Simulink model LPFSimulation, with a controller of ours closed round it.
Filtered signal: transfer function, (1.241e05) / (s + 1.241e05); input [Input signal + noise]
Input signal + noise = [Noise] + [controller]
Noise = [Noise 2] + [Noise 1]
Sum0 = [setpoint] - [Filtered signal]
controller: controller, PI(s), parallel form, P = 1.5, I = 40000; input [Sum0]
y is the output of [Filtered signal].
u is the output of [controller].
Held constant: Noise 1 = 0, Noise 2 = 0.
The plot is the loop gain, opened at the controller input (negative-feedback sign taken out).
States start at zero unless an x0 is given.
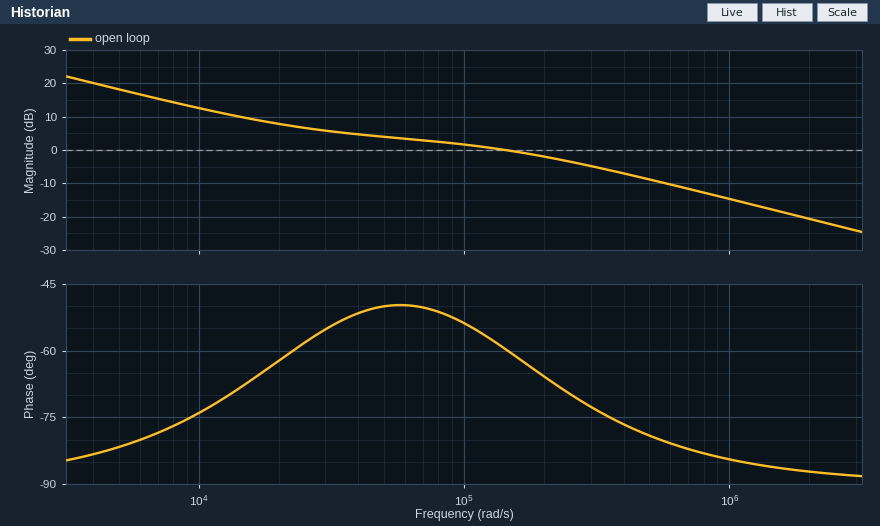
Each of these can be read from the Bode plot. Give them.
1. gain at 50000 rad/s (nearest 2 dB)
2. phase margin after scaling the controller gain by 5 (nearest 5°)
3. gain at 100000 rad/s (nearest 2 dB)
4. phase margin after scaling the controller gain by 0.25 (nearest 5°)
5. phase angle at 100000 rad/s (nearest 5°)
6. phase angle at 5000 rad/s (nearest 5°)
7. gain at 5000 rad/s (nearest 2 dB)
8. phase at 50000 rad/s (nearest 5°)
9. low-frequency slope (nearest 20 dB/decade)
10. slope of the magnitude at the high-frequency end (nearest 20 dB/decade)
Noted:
4 dB
95°
2 dB
105°
-55°
-80°
18 dB
-50°
-20 dB/decade
-20 dB/decade
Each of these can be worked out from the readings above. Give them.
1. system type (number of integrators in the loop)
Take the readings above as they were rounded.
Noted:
1
